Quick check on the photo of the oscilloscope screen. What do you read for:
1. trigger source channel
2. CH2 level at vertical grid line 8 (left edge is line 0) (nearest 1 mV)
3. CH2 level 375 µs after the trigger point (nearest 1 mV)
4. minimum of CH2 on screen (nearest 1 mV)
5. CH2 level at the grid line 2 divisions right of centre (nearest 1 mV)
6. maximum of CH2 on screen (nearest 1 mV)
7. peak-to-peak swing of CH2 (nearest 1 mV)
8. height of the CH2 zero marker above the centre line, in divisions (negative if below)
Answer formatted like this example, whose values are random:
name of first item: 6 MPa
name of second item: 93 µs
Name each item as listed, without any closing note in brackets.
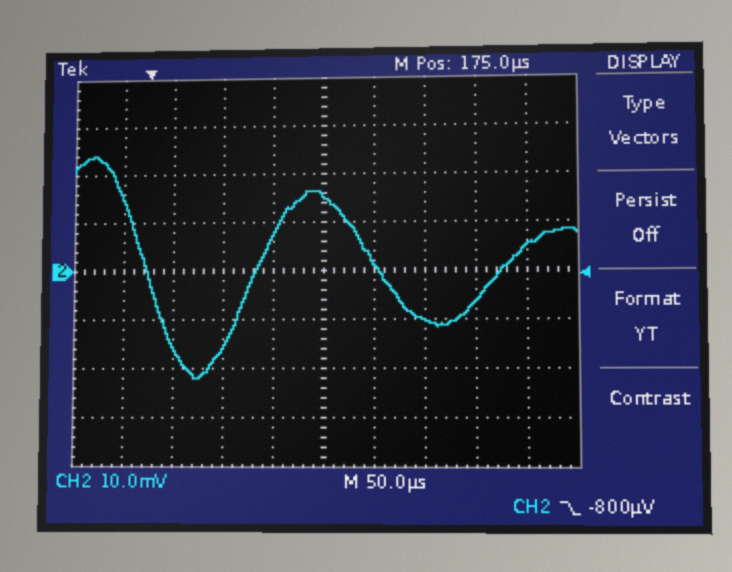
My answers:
trigger source channel: CH2
CH2 level at vertical grid line 8 (left edge is line 0): -6 mV
CH2 level 375 µs after the trigger point: 5 mV
minimum of CH2 on screen: -22 mV
CH2 level at the grid line 2 divisions right of centre: -10 mV
maximum of CH2 on screen: 24 mV
peak-to-peak swing of CH2: 46 mV
height of the CH2 zero marker above the centre line, in divisions: 0.0 div
